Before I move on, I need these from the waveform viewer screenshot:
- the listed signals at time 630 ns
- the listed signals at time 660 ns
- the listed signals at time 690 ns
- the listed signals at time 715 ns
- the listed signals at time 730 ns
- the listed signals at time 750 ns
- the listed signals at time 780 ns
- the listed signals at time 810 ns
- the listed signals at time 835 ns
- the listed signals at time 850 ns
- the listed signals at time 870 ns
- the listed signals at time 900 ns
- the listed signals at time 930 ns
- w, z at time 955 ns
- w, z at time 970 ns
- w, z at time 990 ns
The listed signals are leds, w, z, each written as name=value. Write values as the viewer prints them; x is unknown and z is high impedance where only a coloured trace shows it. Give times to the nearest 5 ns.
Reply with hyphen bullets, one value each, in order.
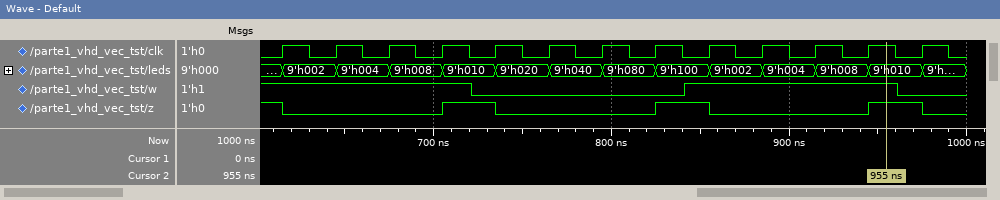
- leds=9'h002, w=1, z=0
- leds=9'h004, w=1, z=0
- leds=9'h008, w=1, z=0
- leds=9'h010, w=1, z=1
- leds=9'h010, w=0, z=1
- leds=9'h020, w=0, z=0
- leds=9'h040, w=0, z=0
- leds=9'h080, w=0, z=0
- leds=9'h100, w=0, z=1
- leds=9'h100, w=1, z=1
- leds=9'h002, w=1, z=0
- leds=9'h004, w=1, z=0
- leds=9'h008, w=1, z=0
- w=1, z=1
- w=0, z=1
- w=0, z=0
